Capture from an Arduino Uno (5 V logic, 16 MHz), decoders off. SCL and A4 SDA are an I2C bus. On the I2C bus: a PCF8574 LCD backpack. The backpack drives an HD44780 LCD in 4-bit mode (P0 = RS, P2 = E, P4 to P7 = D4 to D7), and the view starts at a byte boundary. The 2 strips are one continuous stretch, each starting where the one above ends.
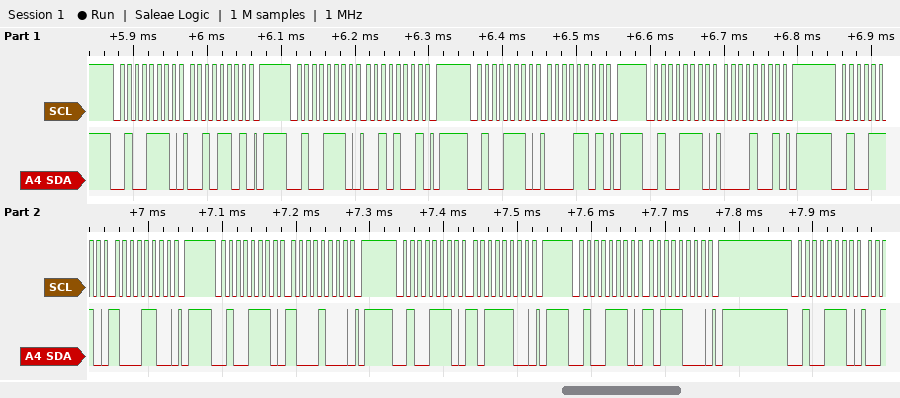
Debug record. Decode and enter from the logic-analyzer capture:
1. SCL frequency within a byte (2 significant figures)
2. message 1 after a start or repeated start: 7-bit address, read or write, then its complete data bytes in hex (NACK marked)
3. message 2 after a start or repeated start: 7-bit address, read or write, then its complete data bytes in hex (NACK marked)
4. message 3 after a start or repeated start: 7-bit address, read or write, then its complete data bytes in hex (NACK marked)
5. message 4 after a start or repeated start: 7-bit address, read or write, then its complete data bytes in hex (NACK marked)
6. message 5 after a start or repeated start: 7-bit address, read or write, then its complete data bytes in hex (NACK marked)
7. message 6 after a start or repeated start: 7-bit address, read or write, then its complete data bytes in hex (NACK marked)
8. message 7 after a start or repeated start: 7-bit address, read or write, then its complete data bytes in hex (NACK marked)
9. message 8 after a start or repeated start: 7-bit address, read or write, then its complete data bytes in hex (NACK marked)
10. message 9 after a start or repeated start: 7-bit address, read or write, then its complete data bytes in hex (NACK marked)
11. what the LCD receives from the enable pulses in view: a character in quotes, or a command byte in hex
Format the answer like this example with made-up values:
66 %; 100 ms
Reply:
100 kHz; 0x27 write: 2D; 0x27 write: 29; 0x27 write: 0D; 0x27 write: 09; 0x27 write: 8C; 0x27 write: 88; 0x27 write: BC; 0x27 write: B8; 0x27 write; ' ' 0x8B
